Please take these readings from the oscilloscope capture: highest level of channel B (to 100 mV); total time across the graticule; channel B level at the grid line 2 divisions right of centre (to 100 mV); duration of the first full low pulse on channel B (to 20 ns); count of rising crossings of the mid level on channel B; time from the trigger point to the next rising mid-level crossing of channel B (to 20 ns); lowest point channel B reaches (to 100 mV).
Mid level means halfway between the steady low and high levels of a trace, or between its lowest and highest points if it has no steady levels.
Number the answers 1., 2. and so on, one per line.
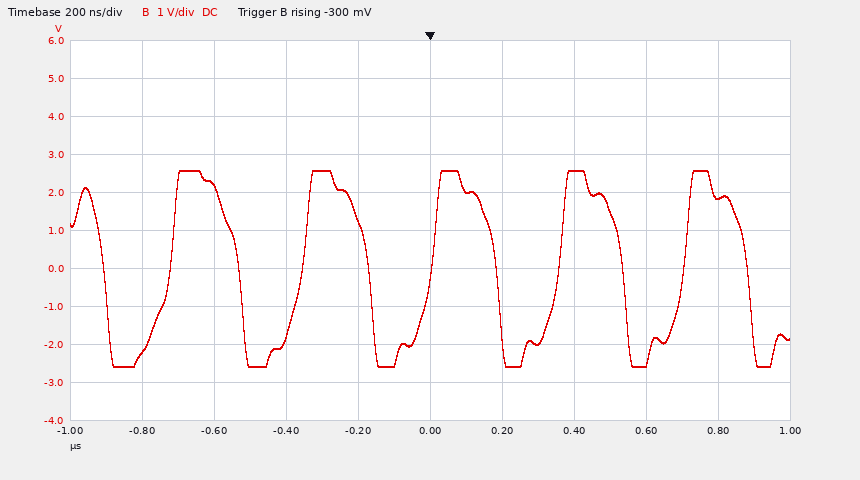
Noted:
1. 2.6 V
2. 2 µs
3. 2.6 V
4. 180 ns
5. 5
6. 360 ns
7. -2.6 V
